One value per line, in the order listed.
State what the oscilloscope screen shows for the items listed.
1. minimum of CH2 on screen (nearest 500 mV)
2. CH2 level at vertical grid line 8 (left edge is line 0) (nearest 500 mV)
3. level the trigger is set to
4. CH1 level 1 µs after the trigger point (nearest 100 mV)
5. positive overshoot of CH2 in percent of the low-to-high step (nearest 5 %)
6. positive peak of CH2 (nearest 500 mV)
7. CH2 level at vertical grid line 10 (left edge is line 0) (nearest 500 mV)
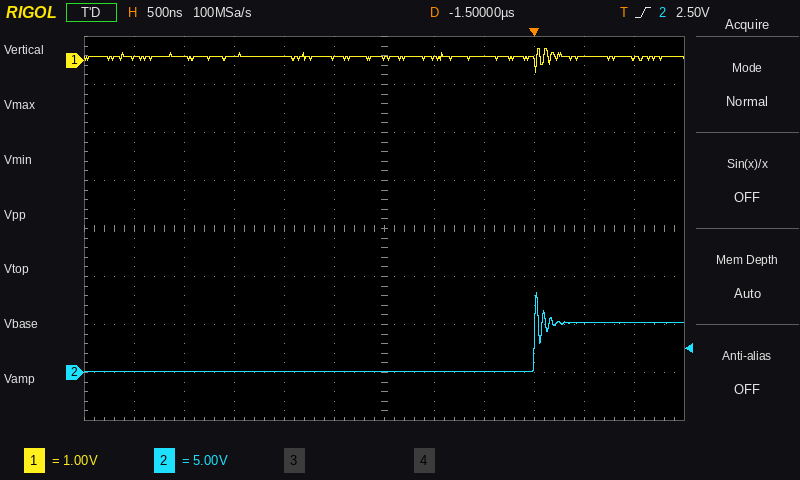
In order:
0.0 V
0.0 V
2.50 V
0.0 V
60 %
8.5 V
5.0 V
